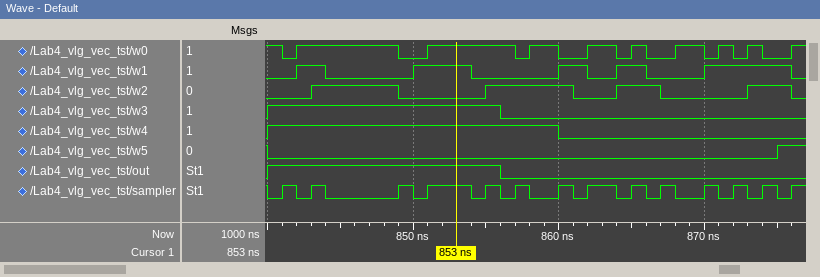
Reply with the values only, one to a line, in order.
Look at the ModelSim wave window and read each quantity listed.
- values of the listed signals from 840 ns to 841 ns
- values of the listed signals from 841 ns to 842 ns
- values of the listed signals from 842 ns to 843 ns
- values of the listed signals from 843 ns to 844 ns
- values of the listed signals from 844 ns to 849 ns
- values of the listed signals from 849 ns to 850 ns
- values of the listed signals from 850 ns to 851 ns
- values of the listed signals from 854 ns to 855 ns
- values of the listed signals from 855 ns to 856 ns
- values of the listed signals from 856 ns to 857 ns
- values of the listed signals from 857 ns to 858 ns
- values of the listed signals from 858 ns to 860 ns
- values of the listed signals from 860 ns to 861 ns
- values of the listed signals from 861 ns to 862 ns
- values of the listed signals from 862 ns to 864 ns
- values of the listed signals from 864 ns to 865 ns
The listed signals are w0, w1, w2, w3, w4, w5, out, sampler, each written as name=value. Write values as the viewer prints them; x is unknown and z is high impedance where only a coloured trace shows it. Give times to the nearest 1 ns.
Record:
w0=1, w1=0, w2=0, w3=1, w4=1, w5=0, out=1, sampler=0
w0=0, w1=0, w2=0, w3=1, w4=1, w5=0, out=1, sampler=1
w0=1, w1=1, w2=0, w3=1, w4=1, w5=0, out=1, sampler=0
w0=1, w1=1, w2=1, w3=1, w4=1, w5=0, out=1, sampler=1
w0=1, w1=0, w2=1, w3=1, w4=1, w5=0, out=1, sampler=0
w0=0, w1=0, w2=0, w3=1, w4=1, w5=0, out=1, sampler=1
w0=0, w1=1, w2=0, w3=1, w4=1, w5=0, out=1, sampler=0
w0=1, w1=0, w2=0, w3=1, w4=1, w5=0, out=1, sampler=0
w0=1, w1=0, w2=1, w3=1, w4=1, w5=0, out=1, sampler=1
w0=1, w1=0, w2=1, w3=0, w4=1, w5=0, out=0, sampler=0
w0=0, w1=0, w2=1, w3=0, w4=1, w5=0, out=0, sampler=1
w0=1, w1=0, w2=1, w3=0, w4=1, w5=0, out=0, sampler=0
w0=0, w1=1, w2=1, w3=0, w4=0, w5=0, out=0, sampler=1
w0=0, w1=1, w2=0, w3=0, w4=0, w5=0, out=0, sampler=0
w0=1, w1=0, w2=0, w3=0, w4=0, w5=0, out=0, sampler=1
w0=0, w1=1, w2=1, w3=0, w4=0, w5=0, out=0, sampler=0
